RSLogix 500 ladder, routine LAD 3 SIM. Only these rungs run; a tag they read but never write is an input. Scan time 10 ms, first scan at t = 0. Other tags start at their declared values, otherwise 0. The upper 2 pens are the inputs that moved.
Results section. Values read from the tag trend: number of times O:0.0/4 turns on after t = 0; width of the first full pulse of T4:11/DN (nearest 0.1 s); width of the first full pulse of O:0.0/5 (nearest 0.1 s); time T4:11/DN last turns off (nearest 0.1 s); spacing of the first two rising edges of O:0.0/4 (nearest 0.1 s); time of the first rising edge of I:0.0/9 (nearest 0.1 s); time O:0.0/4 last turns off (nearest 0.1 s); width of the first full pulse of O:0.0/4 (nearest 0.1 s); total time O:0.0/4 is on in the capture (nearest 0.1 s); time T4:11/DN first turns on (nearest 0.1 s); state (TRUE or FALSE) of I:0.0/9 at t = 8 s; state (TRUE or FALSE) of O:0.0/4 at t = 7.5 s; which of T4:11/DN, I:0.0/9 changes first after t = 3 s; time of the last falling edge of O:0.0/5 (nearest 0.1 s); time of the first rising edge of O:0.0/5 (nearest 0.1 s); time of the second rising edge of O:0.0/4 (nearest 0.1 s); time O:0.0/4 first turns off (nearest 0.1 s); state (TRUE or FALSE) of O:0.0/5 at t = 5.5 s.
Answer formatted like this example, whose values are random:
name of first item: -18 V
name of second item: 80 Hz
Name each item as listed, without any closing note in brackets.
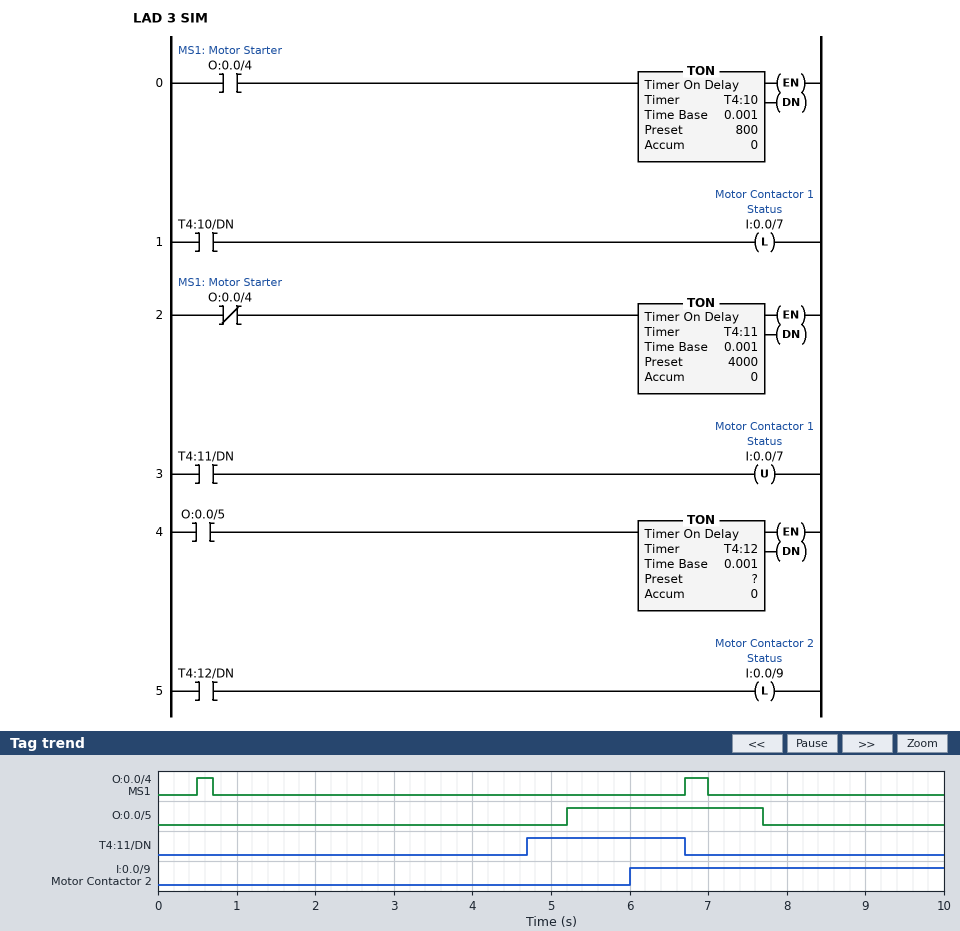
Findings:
number of times O:0.0/4 turns on after t = 0: 2
width of the first full pulse of T4:11/DN: 2.0 s
width of the first full pulse of O:0.0/5: 2.5 s
time T4:11/DN last turns off: 6.7 s
spacing of the first two rising edges of O:0.0/4: 6.2 s
time of the first rising edge of I:0.0/9: 6.0 s
time O:0.0/4 last turns off: 7.0 s
width of the first full pulse of O:0.0/4: 0.2 s
total time O:0.0/4 is on in the capture: 0.5 s
time T4:11/DN first turns on: 4.7 s
state (TRUE or FALSE) of I:0.0/9 at t = 8 s: TRUE
state (TRUE or FALSE) of O:0.0/4 at t = 7.5 s: FALSE
which of T4:11/DN, I:0.0/9 changes first after t = 3 s: T4:11/DN
time of the last falling edge of O:0.0/5: 7.7 s
time of the first rising edge of O:0.0/5: 5.2 s
time of the second rising edge of O:0.0/4: 6.7 s
time O:0.0/4 first turns off: 0.7 s
state (TRUE or FALSE) of O:0.0/5 at t = 5.5 s: TRUE
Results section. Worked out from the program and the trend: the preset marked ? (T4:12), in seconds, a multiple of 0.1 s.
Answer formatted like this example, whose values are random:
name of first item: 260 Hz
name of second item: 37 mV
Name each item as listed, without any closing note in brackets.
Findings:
the preset marked ? (T4:12), in seconds, a multiple of 0.1 s: 0.8 s
